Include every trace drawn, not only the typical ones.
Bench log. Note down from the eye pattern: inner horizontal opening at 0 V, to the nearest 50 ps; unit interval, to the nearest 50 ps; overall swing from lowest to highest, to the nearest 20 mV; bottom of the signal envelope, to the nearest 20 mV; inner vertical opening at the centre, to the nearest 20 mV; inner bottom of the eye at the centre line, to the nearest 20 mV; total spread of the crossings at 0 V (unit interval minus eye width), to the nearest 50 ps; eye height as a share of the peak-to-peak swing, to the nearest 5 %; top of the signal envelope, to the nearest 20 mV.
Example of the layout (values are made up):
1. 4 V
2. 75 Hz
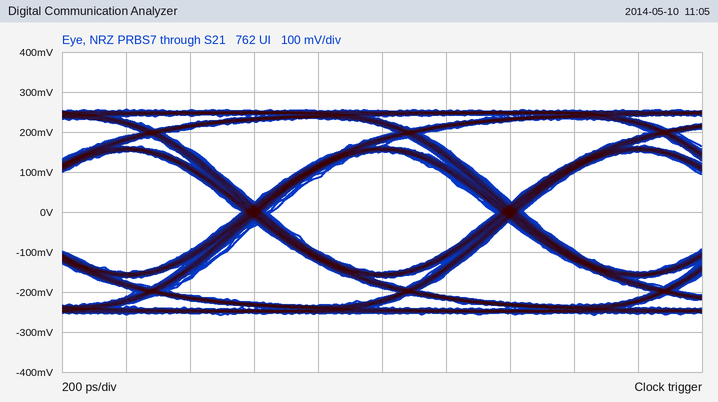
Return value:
1. 700 ps
2. 800 ps
3. 520 mV
4. -260 mV
5. 300 mV
6. -160 mV
7. 100 ps
8. 60 %
9. 260 mV
